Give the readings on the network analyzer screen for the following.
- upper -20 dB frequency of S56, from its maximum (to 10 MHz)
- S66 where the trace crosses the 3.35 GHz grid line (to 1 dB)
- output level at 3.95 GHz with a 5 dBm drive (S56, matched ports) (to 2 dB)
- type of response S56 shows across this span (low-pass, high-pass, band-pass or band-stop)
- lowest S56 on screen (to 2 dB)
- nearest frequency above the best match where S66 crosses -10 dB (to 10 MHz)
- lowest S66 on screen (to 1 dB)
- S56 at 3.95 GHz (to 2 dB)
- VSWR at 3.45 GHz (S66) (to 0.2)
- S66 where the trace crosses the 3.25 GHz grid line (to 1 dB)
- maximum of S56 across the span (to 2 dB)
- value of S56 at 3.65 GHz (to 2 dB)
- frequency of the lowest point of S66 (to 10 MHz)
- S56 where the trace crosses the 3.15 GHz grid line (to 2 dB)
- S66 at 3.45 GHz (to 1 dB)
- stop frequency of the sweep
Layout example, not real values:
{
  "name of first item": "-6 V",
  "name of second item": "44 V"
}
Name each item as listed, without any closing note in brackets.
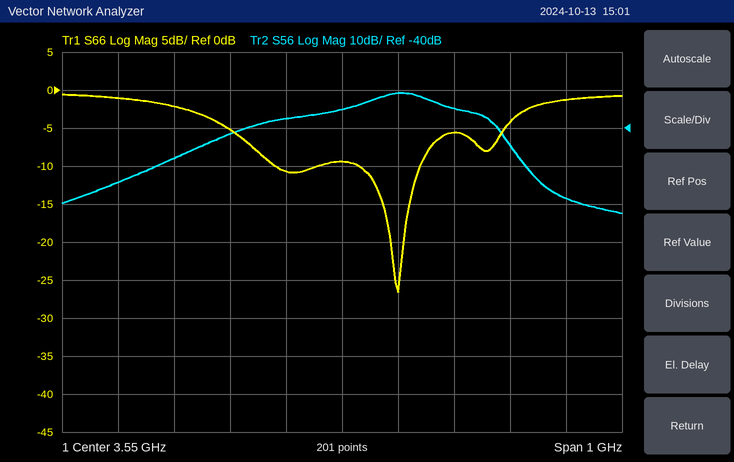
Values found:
{
  "upper -20 dB frequency of S56, from its maximum": "3.88 GHz",
  "S66 where the trace crosses the 3.35 GHz grid line": "-5 dB",
  "output level at 3.95 GHz with a 5 dBm drive (S56, matched ports)": "-54 dBm",
  "type of response S56 shows across this span": "band-pass",
  "lowest S56 on screen": "-62 dB",
  "nearest frequency above the best match where S66 crosses -10 dB": "3.69 GHz",
  "lowest S66 on screen": "-27 dB",
  "S56 at 3.95 GHz": "-58 dB",
  "VSWR at 3.45 GHz (S66)": "1.8",
  "S66 where the trace crosses the 3.25 GHz grid line": "-2 dB",
  "maximum of S56 across the span": "-30 dB",
  "value of S56 at 3.65 GHz": "-30 dB",
  "frequency of the lowest point of S66": "3.65 GHz",
  "S56 where the trace crosses the 3.15 GHz grid line": "-54 dB",
  "S66 at 3.45 GHz": "-11 dB",
  "stop frequency of the sweep": "4.05 GHz"
}
